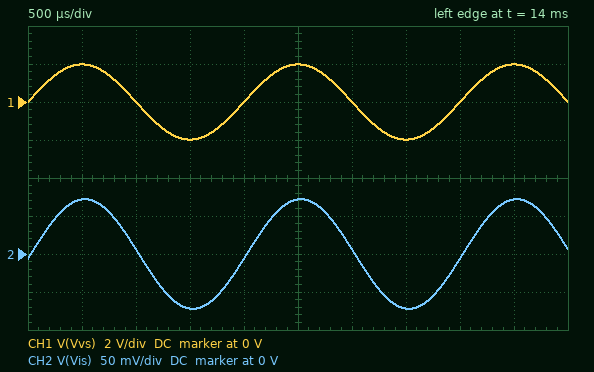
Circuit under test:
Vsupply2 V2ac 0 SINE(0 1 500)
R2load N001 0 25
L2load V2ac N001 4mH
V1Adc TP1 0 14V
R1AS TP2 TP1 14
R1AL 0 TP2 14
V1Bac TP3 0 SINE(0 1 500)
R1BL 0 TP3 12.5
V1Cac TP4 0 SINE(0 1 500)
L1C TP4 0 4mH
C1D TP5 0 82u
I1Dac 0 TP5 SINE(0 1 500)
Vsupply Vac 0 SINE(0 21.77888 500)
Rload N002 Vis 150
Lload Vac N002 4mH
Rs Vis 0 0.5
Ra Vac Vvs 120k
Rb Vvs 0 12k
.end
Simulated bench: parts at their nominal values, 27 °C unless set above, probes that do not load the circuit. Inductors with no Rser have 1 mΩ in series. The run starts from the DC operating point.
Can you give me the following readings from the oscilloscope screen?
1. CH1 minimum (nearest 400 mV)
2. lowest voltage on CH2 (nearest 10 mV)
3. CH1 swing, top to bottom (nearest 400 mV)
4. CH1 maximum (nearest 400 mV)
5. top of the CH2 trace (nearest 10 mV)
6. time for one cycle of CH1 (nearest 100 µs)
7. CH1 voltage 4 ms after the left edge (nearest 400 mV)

-2.0 V
-70 mV
4.0 V
2.0 V
70 mV
2.0 ms
0 V
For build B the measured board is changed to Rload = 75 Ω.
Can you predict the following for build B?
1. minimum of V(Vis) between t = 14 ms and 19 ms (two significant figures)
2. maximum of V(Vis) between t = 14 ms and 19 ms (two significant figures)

-140 mV
140 mV
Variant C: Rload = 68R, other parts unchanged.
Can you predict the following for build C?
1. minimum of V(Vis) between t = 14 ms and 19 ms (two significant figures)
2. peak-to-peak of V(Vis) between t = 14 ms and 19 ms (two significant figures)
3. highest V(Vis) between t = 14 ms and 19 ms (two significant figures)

-160 mV
310 mV
160 mV
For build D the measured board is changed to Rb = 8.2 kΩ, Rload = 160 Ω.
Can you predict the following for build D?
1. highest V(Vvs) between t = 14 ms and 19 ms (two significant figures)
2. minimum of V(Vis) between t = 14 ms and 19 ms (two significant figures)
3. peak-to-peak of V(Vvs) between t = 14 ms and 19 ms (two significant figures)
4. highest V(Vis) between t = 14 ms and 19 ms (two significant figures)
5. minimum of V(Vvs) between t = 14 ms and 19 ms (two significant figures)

1.4 V
-68 mV
2.8 V
68 mV
-1.4 V
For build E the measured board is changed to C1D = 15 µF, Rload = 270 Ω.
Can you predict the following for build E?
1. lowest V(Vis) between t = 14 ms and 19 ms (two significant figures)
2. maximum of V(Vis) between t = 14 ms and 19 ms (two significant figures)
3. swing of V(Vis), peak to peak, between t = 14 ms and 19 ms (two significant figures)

-40 mV
40 mV
80 mV
